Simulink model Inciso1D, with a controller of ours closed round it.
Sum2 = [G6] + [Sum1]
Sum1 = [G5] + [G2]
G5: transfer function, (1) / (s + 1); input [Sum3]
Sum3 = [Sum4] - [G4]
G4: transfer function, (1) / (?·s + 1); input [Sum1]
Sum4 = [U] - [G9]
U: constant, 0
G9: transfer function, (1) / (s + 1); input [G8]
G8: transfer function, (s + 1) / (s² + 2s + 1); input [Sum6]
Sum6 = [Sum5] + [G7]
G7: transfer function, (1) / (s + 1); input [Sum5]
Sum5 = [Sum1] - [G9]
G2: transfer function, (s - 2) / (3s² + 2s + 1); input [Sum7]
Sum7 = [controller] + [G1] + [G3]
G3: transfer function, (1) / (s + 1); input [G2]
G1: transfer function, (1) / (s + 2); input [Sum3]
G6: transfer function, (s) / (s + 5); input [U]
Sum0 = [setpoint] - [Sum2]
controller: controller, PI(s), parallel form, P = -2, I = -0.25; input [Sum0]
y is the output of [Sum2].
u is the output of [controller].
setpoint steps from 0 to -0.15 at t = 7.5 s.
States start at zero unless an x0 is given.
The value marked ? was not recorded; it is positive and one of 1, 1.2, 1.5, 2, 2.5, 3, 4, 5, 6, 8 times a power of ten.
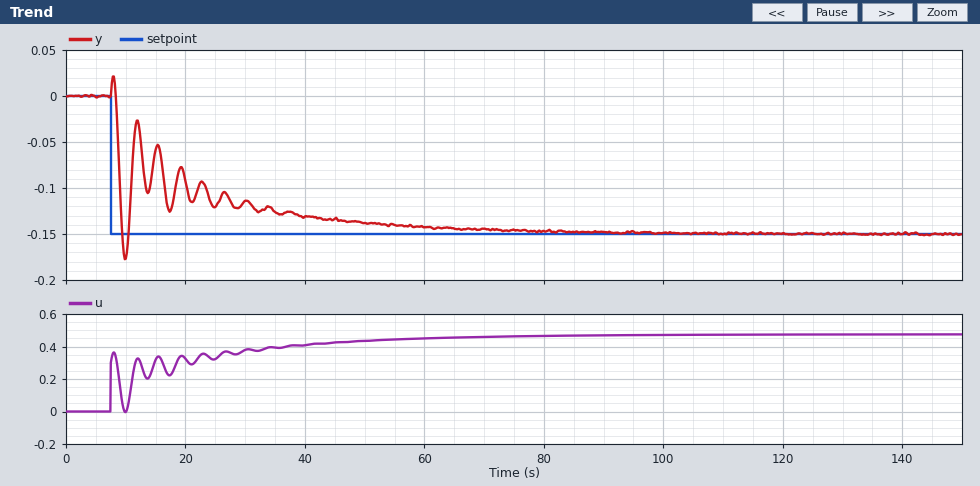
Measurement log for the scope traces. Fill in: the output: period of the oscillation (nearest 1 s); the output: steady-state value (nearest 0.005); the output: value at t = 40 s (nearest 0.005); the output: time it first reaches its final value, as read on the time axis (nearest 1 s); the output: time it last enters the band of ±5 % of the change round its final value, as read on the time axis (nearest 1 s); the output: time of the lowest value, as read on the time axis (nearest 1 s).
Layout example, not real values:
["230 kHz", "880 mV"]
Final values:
["4 s", "-0.150", "-0.130", "9 s", "61 s", "10 s"]
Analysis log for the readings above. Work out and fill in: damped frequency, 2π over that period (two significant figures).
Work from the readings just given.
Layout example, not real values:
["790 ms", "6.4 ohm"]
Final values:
["1.6 rad/s"]
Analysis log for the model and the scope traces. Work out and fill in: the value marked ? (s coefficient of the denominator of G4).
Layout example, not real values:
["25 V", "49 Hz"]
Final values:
["0.5"]
